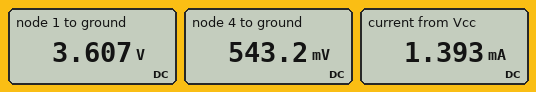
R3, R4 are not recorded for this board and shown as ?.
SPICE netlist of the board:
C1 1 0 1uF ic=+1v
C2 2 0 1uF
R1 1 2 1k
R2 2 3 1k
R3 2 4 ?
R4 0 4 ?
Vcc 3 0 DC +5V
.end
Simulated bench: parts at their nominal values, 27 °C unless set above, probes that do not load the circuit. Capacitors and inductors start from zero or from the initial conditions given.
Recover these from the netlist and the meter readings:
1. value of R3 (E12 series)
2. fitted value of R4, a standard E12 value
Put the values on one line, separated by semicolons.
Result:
2.2 kΩ; 390 Ω
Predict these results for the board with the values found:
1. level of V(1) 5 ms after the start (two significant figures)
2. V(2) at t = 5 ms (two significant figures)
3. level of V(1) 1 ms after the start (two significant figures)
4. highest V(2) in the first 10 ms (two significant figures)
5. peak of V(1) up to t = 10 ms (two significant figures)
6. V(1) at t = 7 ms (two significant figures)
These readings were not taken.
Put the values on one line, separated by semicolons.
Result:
3.3 V; 3.4 V; 1.5 V; 3.6 V; 3.6 V; 3.5 V
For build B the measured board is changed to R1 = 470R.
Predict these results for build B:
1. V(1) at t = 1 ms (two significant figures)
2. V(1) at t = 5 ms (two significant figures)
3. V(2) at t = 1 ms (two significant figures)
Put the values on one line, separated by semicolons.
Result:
1.7 V; 3.4 V; 2.2 V
